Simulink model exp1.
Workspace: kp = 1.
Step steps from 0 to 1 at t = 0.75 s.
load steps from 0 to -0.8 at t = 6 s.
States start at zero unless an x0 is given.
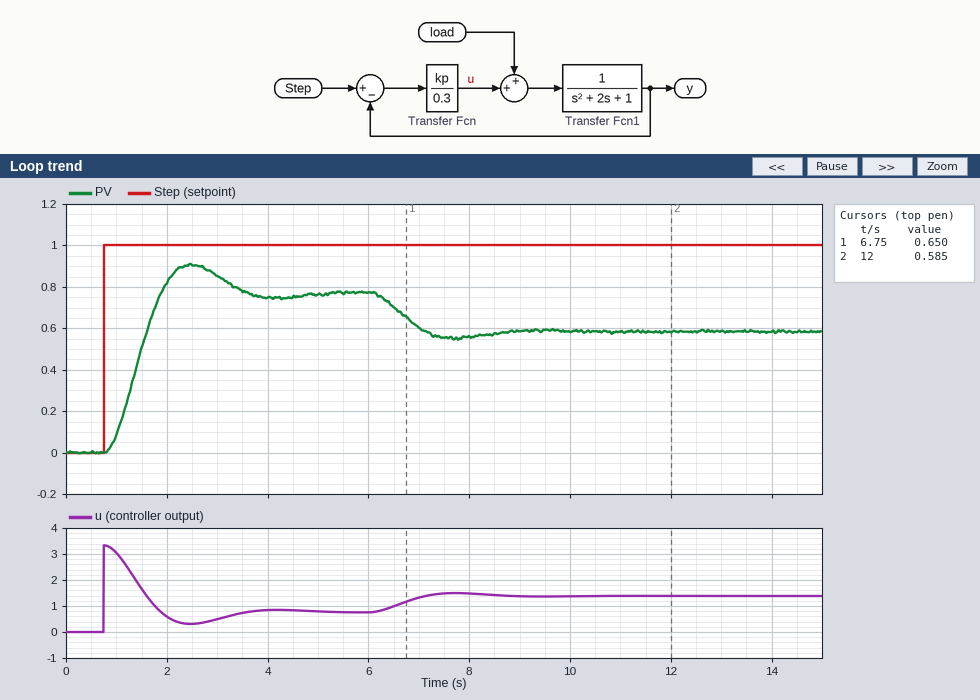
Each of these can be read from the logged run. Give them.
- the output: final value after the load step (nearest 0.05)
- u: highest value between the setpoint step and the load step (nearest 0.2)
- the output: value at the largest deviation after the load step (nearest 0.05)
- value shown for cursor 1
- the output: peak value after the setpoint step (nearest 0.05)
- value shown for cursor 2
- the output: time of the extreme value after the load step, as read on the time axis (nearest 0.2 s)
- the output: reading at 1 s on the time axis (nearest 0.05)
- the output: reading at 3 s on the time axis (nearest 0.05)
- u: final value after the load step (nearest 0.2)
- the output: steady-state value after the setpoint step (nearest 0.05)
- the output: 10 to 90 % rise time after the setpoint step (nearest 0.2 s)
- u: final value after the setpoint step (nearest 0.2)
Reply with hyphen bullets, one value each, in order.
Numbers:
- 0.60
- 3.4
- 0.55
- 0.650
- 0.90
- 0.585
- 7.8 s
- 0.10
- 0.85
- 1.4
- 0.75
- 0.8 s
- 0.8
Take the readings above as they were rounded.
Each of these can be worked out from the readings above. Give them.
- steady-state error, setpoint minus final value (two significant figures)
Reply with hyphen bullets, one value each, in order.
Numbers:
- 0.25
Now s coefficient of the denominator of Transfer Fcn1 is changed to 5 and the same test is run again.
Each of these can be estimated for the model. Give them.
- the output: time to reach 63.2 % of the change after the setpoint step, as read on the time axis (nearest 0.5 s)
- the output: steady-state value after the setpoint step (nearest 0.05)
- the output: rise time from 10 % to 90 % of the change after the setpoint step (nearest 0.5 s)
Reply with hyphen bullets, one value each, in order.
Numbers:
- 2.0 s
- 0.75
- 2.0 s
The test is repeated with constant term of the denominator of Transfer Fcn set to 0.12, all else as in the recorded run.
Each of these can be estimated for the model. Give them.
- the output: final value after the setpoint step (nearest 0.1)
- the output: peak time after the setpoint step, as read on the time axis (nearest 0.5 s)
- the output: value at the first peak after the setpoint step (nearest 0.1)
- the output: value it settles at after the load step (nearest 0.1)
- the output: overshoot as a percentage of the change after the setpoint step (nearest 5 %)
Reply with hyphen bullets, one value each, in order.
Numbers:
- 0.9
- 2.0 s
- 1.2
- 0.8
- 35 %
